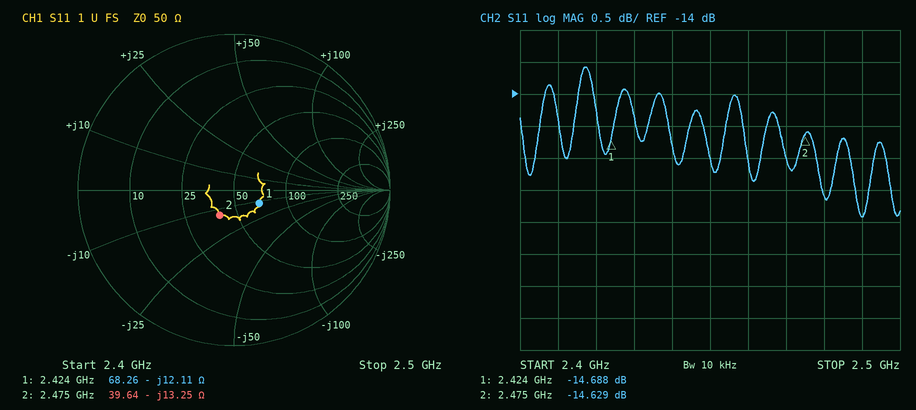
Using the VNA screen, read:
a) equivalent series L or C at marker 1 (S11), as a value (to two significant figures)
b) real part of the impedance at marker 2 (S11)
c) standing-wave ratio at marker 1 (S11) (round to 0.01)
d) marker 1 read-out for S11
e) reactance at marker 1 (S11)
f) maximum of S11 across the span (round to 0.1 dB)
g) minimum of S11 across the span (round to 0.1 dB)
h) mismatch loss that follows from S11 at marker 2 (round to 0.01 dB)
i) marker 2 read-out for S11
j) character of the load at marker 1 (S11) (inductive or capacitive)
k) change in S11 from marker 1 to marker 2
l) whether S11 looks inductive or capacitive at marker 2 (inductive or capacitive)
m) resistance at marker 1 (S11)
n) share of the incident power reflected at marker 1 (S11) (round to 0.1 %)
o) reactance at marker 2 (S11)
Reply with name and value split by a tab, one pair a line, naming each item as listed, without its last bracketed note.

equivalent series L or C at marker 1 (S11), as a value	5.4 pF
real part of the impedance at marker 2	39.64 Ω
standing-wave ratio at marker 1 (S11)	1.45
marker 1 read-out for S11	-14.688 dB
reactance at marker 1	-12.11 Ω
maximum of S11 across the span	-13.6 dB
minimum of S11 across the span	-15.9 dB
mismatch loss that follows from S11 at marker 2	0.15 dB
marker 2 read-out for S11	-14.629 dB
character of the load at marker 1 (S11)	capacitive
change in S11 from marker 1 to marker 2	0.059 dB
whether S11 looks inductive or capacitive at marker 2	capacitive
resistance at marker 1	68.26 Ω
share of the incident power reflected at marker 1 (S11)	3.4 %
reactance at marker 2	-13.25 Ω
